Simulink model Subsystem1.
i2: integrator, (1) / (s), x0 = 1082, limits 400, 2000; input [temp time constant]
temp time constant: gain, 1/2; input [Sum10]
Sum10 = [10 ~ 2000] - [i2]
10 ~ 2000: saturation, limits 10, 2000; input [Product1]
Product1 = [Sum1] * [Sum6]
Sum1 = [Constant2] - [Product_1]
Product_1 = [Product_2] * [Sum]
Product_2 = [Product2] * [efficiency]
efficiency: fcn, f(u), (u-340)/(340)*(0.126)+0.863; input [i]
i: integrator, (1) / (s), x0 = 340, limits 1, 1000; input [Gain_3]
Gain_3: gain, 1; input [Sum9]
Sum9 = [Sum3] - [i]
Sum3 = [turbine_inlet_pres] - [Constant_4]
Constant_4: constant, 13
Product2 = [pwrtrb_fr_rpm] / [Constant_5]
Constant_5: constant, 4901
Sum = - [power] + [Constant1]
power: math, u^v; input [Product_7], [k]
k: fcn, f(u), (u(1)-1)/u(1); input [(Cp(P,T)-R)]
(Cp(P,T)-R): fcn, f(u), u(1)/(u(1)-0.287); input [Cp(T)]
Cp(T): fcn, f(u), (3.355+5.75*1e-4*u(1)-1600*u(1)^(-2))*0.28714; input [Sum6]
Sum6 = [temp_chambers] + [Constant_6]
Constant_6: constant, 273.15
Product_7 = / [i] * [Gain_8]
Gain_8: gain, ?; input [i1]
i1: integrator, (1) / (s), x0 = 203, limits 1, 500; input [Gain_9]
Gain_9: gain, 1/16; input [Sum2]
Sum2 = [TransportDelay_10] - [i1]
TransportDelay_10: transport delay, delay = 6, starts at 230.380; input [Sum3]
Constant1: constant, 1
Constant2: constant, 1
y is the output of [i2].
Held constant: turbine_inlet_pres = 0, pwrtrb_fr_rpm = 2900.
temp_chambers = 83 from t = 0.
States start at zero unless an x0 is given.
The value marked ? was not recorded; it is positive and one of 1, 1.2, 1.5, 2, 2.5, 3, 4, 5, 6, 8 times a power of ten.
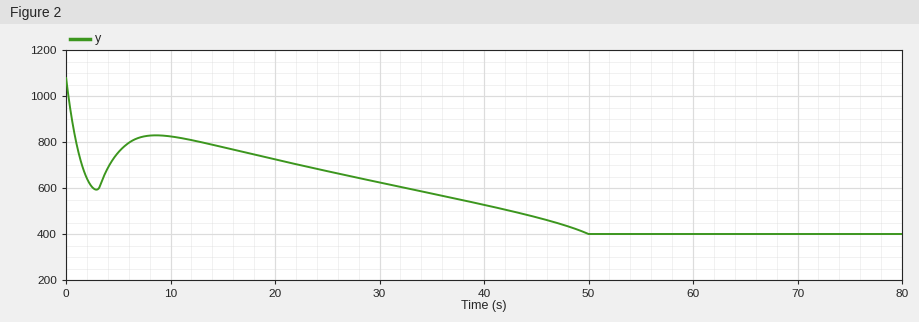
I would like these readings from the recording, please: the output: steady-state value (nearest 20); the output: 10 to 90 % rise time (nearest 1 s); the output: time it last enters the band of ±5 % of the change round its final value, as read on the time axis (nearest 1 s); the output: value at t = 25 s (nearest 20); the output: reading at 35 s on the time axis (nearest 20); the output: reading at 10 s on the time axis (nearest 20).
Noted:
400
45 s
48 s
680
580
820
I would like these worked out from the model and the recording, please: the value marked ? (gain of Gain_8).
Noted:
0.8
